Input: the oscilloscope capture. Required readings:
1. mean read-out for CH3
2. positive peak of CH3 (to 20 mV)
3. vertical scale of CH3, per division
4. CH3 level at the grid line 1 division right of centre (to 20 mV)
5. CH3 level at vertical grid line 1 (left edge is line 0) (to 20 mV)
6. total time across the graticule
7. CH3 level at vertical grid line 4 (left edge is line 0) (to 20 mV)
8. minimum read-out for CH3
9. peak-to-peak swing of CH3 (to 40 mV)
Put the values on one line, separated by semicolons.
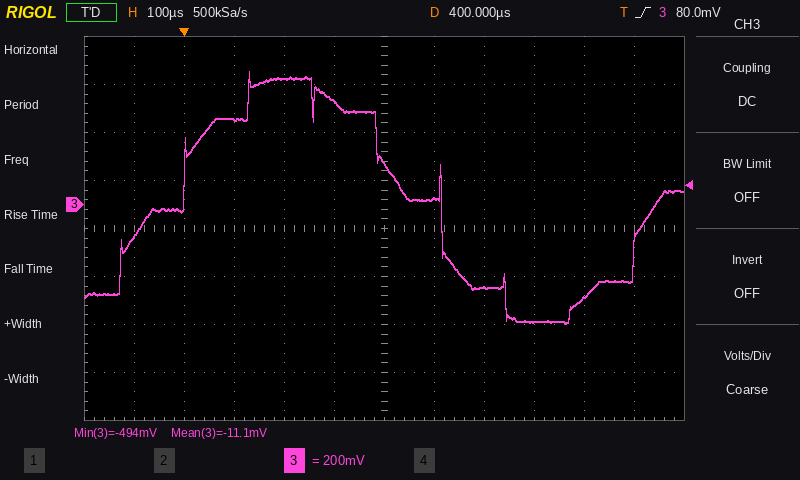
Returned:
-11.1 mV; 560 mV; 200 mV; 20 mV; -140 mV; 1.2 ms; 520 mV; -494 mV; 1.04 V
